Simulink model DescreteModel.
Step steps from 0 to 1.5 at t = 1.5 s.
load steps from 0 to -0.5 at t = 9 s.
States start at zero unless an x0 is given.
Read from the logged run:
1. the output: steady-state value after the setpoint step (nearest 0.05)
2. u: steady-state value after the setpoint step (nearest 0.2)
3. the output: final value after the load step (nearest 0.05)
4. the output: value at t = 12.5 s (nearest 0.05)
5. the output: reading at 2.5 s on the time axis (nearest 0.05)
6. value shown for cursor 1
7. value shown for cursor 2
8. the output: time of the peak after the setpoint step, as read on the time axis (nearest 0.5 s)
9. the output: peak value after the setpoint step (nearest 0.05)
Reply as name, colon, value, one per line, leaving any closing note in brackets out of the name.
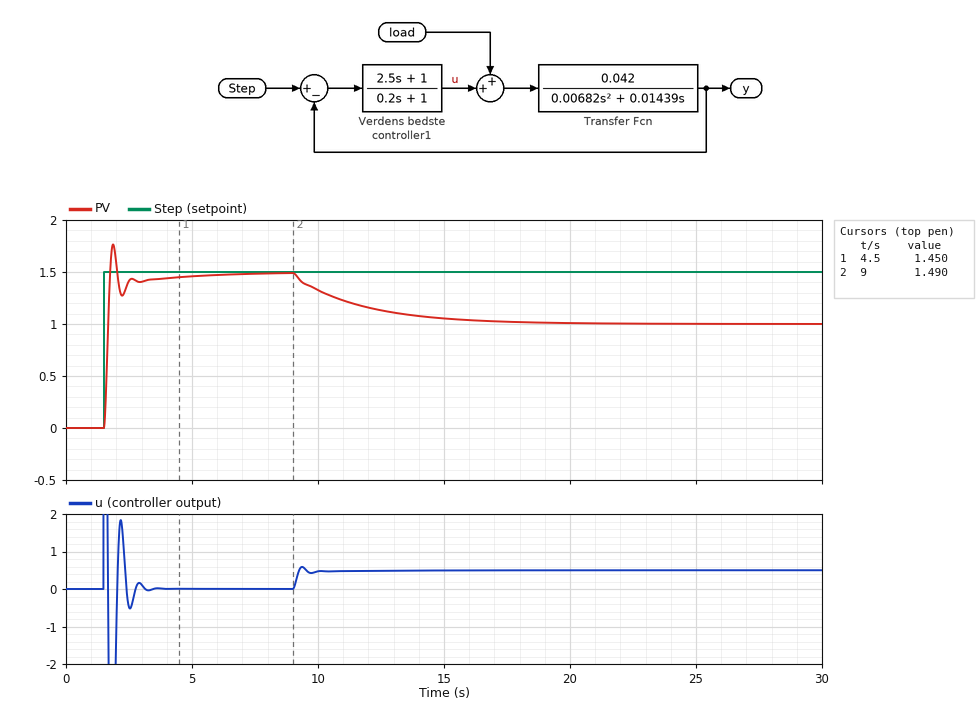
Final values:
the output: steady-state value after the setpoint step: 1.50
u: steady-state value after the setpoint step: 0.0
the output: final value after the load step: 1.00
the output: value at t = 12.5 s: 1.15
the output: reading at 2.5 s on the time axis: 1.40
value shown for cursor 1: 1.450
value shown for cursor 2: 1.490
the output: time of the peak after the setpoint step, as read on the time axis: 2.0 s
the output: peak value after the setpoint step: 1.75
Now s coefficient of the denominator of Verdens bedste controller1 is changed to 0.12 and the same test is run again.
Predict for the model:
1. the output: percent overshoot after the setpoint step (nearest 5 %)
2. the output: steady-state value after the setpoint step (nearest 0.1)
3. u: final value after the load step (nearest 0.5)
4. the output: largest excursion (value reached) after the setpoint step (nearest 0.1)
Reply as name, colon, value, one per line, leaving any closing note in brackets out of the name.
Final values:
the output: percent overshoot after the setpoint step: 10 %
the output: steady-state value after the setpoint step: 1.5
u: final value after the load step: 0.5
the output: largest excursion (value reached) after the setpoint step: 1.7
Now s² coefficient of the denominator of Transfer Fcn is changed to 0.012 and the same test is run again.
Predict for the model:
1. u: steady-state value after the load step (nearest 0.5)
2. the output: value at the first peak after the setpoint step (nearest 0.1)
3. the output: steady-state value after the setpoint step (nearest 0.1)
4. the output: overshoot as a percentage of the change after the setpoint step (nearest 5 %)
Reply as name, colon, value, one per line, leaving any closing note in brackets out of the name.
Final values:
u: steady-state value after the load step: 0.5
the output: value at the first peak after the setpoint step: 1.7
the output: steady-state value after the setpoint step: 1.5
the output: overshoot as a percentage of the change after the setpoint step: 15 %
